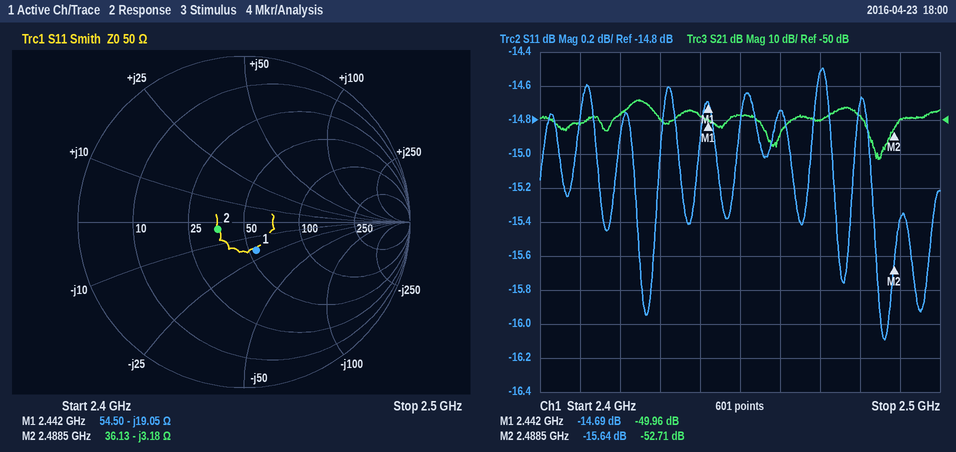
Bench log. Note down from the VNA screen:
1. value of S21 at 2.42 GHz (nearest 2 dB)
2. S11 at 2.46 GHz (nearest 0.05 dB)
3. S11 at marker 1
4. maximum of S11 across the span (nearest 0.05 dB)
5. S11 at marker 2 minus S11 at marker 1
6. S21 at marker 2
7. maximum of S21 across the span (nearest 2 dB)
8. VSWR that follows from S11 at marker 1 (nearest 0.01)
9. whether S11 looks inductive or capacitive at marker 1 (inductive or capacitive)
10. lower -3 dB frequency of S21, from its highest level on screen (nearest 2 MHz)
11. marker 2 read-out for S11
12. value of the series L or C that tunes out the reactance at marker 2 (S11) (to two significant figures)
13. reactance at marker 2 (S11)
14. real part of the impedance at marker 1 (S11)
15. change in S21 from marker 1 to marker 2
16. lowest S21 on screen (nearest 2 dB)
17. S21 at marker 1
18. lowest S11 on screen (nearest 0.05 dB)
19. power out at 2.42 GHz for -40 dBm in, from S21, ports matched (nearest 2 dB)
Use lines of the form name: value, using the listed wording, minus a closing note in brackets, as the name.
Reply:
value of S21 at 2.42 GHz: -48 dB
S11 at 2.46 GHz: -14.75 dB
S11 at marker 1: -14.69 dB
maximum of S11 across the span: -14.50 dB
S11 at marker 2 minus S11 at marker 1: -0.95 dB
S21 at marker 2: -52.71 dB
maximum of S21 across the span: -44 dB
VSWR that follows from S11 at marker 1: 1.45
whether S11 looks inductive or capacitive at marker 1: capacitive
lower -3 dB frequency of S21, from its highest level on screen: 2.422 GHz
marker 2 read-out for S11: -15.64 dB
value of the series L or C that tunes out the reactance at marker 2 (S11): 200 pH
reactance at marker 2: -3.18 Ω
real part of the impedance at marker 1: 54.50 Ω
change in S21 from marker 1 to marker 2: -2.75 dB
lowest S21 on screen: -62 dB
S21 at marker 1: -49.96 dB
lowest S11 on screen: -16.10 dB
power out at 2.42 GHz for -40 dBm in, from S21, ports matched: -88 dBm
